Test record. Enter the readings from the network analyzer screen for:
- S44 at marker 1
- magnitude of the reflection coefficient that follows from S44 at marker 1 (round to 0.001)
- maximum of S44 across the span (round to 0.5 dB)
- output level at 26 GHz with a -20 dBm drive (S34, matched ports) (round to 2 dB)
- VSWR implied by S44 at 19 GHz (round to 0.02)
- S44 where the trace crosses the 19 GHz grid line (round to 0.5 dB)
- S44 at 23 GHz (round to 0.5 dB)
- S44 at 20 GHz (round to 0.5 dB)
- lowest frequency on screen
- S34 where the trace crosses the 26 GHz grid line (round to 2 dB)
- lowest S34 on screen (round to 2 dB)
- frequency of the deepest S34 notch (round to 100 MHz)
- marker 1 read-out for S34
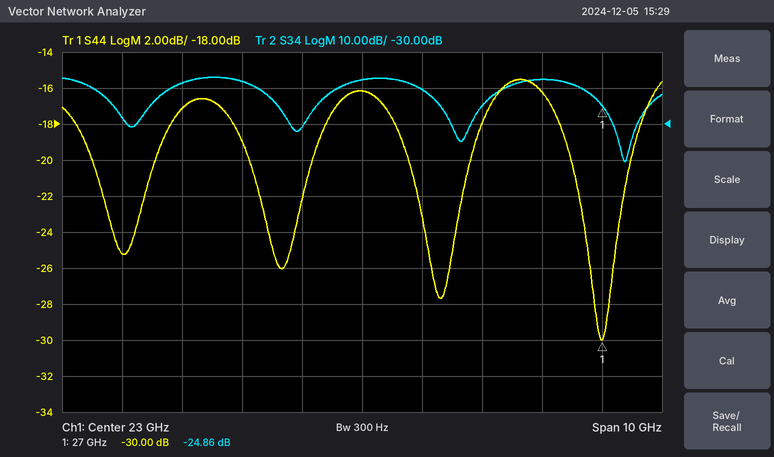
-30.00 dB
0.032
-15.5 dB
-38 dBm
1.12
-25.0 dB
-16.0 dB
-17.0 dB
18 GHz
-18 dB
-40 dB
27.4 GHz
-24.86 dB
